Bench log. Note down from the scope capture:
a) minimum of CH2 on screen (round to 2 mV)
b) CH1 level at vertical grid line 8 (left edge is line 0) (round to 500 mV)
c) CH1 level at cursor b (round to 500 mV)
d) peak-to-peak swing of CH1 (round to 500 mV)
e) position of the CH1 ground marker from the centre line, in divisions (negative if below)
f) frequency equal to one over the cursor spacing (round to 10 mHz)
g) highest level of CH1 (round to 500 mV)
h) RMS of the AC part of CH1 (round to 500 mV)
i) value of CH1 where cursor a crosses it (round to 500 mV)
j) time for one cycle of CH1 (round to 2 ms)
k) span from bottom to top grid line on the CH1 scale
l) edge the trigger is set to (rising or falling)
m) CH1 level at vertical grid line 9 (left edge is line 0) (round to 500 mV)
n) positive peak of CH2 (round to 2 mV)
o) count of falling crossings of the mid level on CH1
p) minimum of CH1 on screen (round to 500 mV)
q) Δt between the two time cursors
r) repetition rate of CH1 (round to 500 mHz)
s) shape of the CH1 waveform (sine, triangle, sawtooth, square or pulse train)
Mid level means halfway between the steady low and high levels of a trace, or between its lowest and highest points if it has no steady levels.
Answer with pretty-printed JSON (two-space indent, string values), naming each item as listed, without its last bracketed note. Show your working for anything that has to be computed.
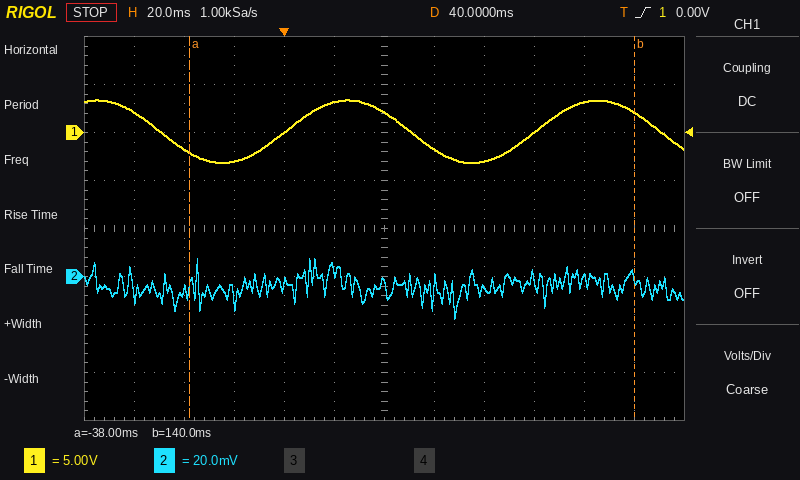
{
  "minimum of CH2 on screen": "-18 mV",
  "CH1 level at vertical grid line 8 (left edge is line 0)": "-3.0 V",
  "CH1 level at cursor b": "2.0 V",
  "peak-to-peak swing of CH1": "3.5 V − (-3.0 V) = 6.5 V",
  "position of the CH1 ground marker from the centre line, in divisions": "+2.0 div",
  "frequency equal to one over the cursor spacing": "1 / 178 ms ≈ 5.62 Hz",
  "highest level of CH1": "3.5 V",
  "RMS of the AC part of CH1": "6.5 V / (2√2) ≈ 2.30 V, so 2.5 V to the nearest 500 mV",
  "value of CH1 where cursor a crosses it": "-2.0 V",
  "time for one cycle of CH1": "100 ms",
  "span from bottom to top grid line on the CH1 scale": "40 V",
  "edge the trigger is set to": "rising",
  "CH1 level at vertical grid line 9 (left edge is line 0)": "0.0 V",
  "positive peak of CH2": "8 mV",
  "count of falling crossings of the mid level on CH1": "3",
  "minimum of CH1 on screen": "-3.0 V",
  "Δt between the two time cursors": "140 ms − (-38 ms) = 178 ms",
  "repetition rate of CH1": "1 / 100 ms ≈ 10.0 Hz",
  "shape of the CH1 waveform": "sine"
}
